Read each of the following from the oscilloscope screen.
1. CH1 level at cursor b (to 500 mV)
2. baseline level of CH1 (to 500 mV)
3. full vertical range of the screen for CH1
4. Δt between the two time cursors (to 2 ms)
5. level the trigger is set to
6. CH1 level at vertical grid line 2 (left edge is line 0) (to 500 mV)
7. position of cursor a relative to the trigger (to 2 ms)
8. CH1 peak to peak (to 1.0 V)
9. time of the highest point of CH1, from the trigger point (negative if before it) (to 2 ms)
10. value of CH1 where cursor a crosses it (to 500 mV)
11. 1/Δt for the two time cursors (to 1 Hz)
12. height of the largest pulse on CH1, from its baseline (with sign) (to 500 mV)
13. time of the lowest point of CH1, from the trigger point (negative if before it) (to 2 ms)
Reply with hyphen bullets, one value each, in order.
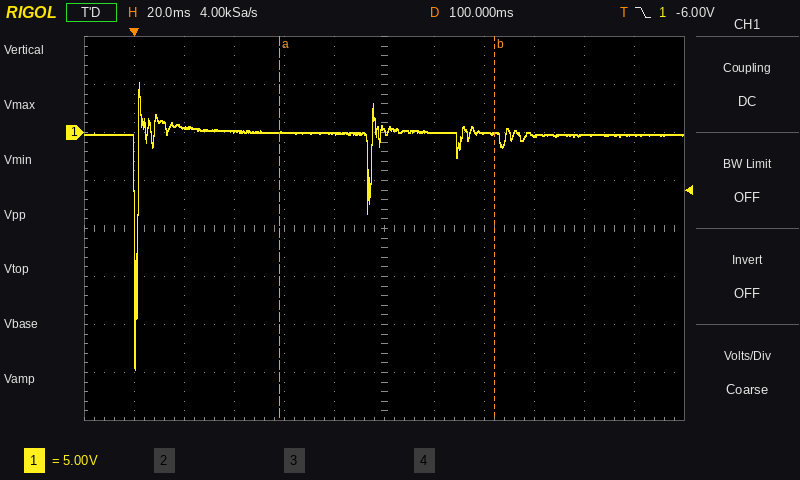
- 0.0 V
- 0.0 V
- 40 V
- 86 ms
- -6.00 V
- 500 mV
- +58 ms
- 30.0 V
- +2 ms
- 0.0 V
- 12 Hz
- -24.5 V
- 0 ms
